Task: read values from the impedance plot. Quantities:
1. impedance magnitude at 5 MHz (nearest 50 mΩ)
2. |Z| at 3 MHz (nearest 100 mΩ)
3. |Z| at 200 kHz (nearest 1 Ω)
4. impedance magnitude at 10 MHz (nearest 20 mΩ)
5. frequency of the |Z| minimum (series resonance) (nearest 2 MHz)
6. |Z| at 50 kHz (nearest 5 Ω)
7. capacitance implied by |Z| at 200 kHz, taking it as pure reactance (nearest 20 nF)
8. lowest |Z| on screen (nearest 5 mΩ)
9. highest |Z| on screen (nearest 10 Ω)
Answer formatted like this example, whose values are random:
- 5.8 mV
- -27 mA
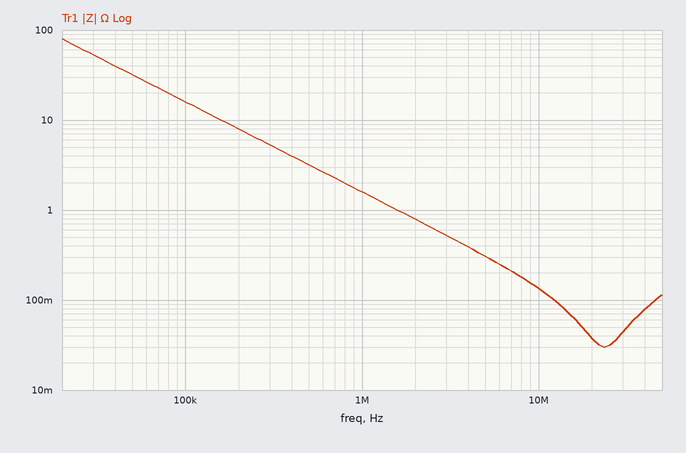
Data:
- 300 mΩ
- 500 mΩ
- 8 Ω
- 140 mΩ
- 24 MHz
- 30 Ω
- 100 nF
- 30 mΩ
- 80 Ω
